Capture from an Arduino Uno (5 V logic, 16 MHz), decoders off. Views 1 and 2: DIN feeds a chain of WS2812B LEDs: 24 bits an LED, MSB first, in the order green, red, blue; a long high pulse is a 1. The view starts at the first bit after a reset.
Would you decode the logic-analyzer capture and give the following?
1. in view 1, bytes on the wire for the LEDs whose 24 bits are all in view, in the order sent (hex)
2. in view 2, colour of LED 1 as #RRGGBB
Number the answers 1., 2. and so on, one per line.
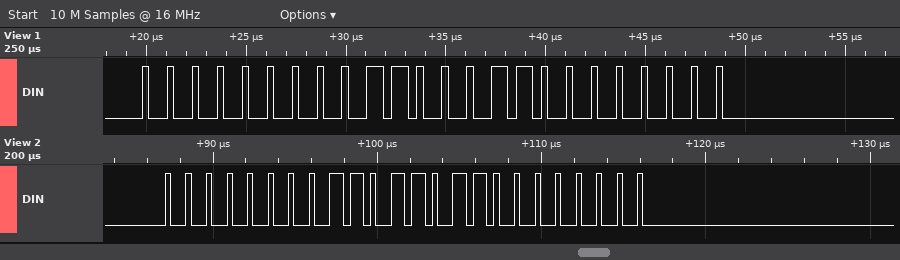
1. 00 63 00
2. #DB0000
